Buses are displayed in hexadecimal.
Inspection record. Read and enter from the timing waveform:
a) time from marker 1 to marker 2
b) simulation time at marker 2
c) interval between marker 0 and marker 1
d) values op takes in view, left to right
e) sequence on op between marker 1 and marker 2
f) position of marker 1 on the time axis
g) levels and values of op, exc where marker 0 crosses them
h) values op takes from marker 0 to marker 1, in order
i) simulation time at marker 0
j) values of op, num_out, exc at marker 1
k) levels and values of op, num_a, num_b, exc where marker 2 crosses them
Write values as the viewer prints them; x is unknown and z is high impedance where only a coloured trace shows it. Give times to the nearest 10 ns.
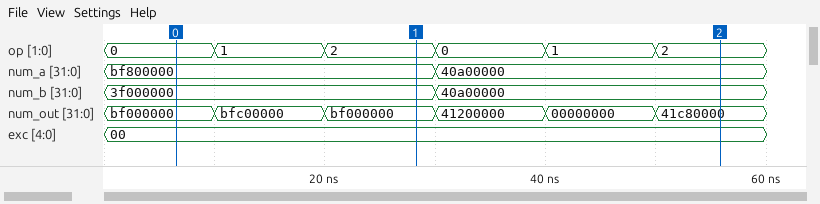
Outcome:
30 ns
60 ns
20 ns
0, 1, 2, 0, 1, 2
2, 0, 1, 2
30 ns
op=0, exc=00
0, 1, 2
10 ns
op=2, num_out=bf000000, exc=00
op=2, num_a=40a00000, num_b=40a00000, exc=00
